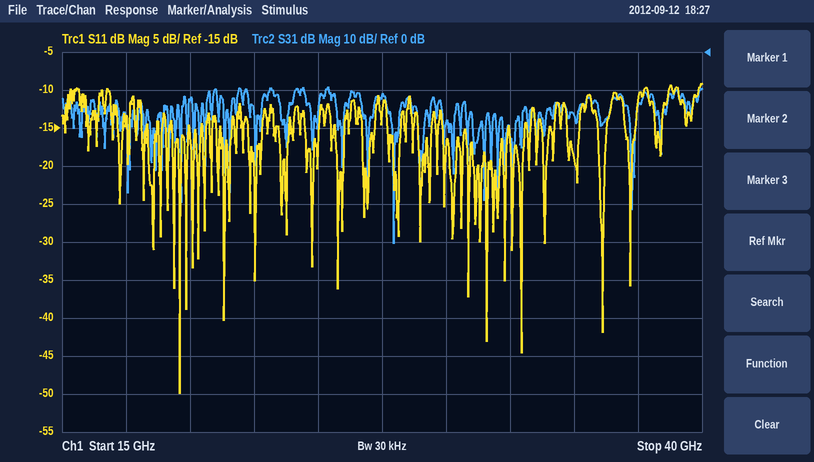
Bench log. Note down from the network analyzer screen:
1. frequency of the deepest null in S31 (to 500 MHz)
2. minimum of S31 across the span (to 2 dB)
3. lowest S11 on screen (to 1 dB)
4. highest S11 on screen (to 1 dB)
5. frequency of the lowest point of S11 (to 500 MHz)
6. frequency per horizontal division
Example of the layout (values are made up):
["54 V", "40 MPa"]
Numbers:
["28.0 GHz", "-50 dB", "-50 dB", "-9 dB", "19.5 GHz", "2.5 GHz"]
